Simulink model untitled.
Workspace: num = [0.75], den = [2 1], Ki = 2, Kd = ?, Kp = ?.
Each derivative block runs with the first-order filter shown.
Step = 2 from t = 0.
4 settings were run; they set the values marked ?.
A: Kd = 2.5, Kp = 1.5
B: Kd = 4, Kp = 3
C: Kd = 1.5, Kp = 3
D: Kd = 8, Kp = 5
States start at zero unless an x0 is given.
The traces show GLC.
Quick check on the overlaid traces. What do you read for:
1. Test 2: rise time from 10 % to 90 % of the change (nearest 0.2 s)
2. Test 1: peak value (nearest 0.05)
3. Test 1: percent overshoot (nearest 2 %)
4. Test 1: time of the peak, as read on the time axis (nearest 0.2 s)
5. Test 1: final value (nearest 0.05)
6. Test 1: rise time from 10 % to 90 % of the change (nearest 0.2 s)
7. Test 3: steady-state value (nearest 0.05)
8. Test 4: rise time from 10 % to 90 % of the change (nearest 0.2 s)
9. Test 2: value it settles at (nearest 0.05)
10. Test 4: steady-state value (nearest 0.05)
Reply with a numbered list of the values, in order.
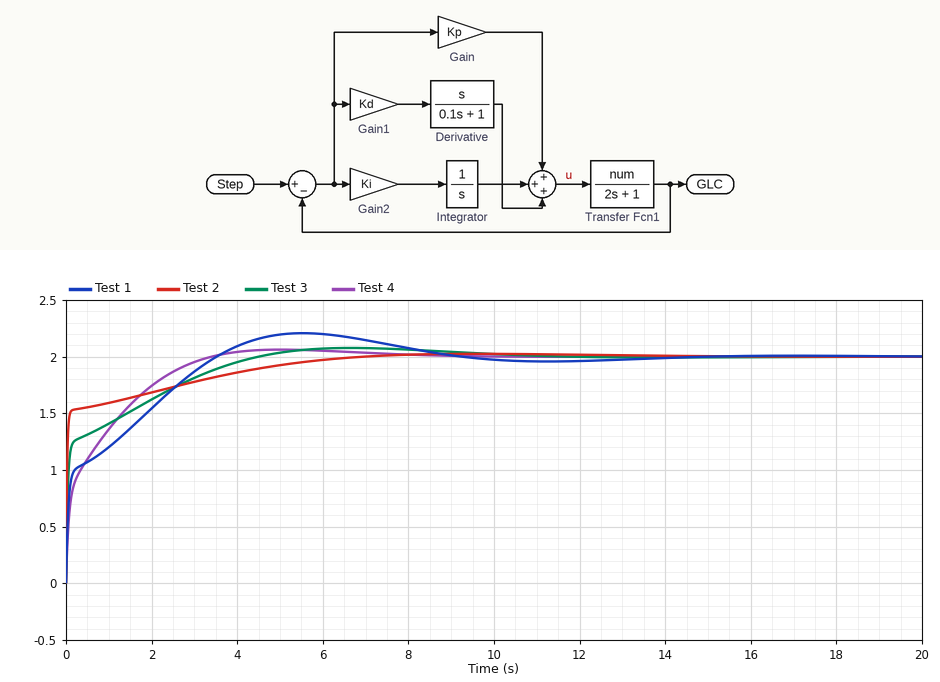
1. 3.2 s
2. 2.20
3. 10 %
4. 5.6 s
5. 2.00
6. 2.8 s
7. 2.00
8. 2.2 s
9. 2.00
10. 2.00
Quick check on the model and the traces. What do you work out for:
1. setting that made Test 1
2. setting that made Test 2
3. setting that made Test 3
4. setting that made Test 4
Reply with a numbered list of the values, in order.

1. A
2. D
3. B
4. C
